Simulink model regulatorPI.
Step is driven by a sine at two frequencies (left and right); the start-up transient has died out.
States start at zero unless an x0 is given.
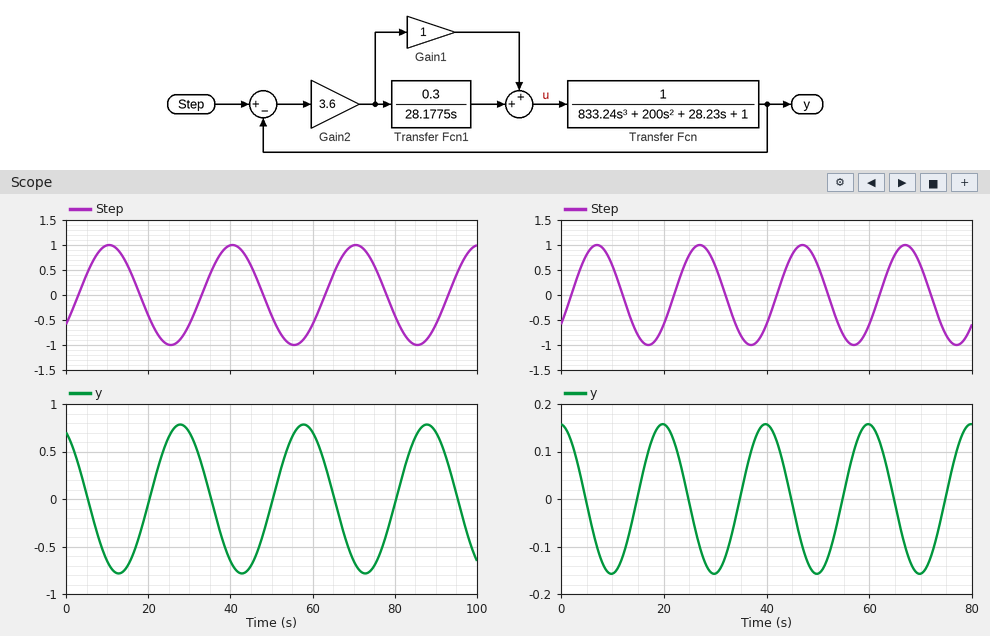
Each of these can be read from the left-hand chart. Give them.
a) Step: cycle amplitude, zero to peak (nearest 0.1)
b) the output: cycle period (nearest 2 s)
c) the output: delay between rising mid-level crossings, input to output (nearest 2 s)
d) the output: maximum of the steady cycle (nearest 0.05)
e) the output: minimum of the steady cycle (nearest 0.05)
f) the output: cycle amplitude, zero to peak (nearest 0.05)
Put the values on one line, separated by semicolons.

1.0; 30 s; 18 s; 0.80; -0.80; 0.80
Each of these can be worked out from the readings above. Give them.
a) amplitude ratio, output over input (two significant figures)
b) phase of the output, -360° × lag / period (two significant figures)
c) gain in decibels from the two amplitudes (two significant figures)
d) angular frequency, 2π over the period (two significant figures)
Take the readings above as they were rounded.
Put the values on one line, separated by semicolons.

0.80; -220°; -1.9 dB; 0.21 rad/s
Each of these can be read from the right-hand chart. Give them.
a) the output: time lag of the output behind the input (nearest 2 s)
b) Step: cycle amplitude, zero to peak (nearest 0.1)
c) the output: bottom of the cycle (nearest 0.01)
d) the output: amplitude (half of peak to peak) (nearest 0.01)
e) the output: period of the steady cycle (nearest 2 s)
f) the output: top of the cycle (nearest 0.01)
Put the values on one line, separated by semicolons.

12 s; 1.0; -0.16; 0.16; 20 s; 0.16
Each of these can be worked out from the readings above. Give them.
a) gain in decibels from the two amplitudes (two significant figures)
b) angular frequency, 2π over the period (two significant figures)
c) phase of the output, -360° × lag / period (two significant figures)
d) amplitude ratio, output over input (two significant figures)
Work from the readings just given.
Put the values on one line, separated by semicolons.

-16 dB; 0.31 rad/s; -220°; 0.16
